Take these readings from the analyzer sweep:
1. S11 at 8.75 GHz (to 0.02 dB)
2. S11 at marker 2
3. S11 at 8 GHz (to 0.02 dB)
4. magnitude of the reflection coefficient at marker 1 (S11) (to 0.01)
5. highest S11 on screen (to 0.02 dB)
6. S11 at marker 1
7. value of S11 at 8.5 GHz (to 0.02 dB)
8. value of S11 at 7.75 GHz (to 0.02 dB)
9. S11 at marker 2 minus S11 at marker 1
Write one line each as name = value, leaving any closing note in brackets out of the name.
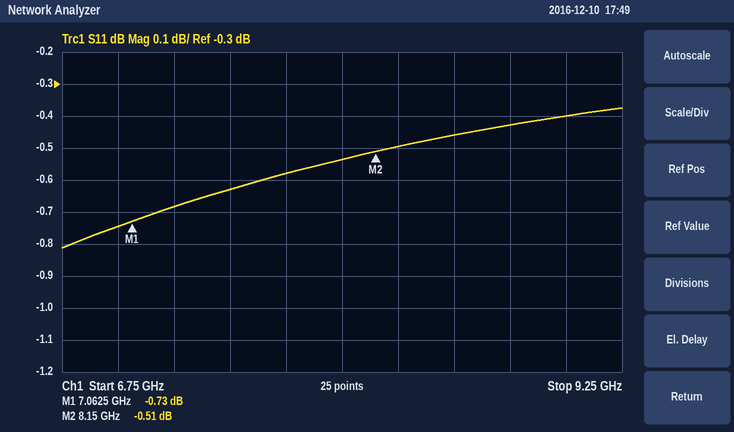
S11 at 8.75 GHz = -0.42 dB
S11 at marker 2 = -0.51 dB
S11 at 8 GHz = -0.54 dB
magnitude of the reflection coefficient at marker 1 (S11) = 0.92
highest S11 on screen = -0.38 dB
S11 at marker 1 = -0.73 dB
value of S11 at 8.5 GHz = -0.46 dB
value of S11 at 7.75 GHz = -0.58 dB
S11 at marker 2 minus S11 at marker 1 = 0.22 dB
